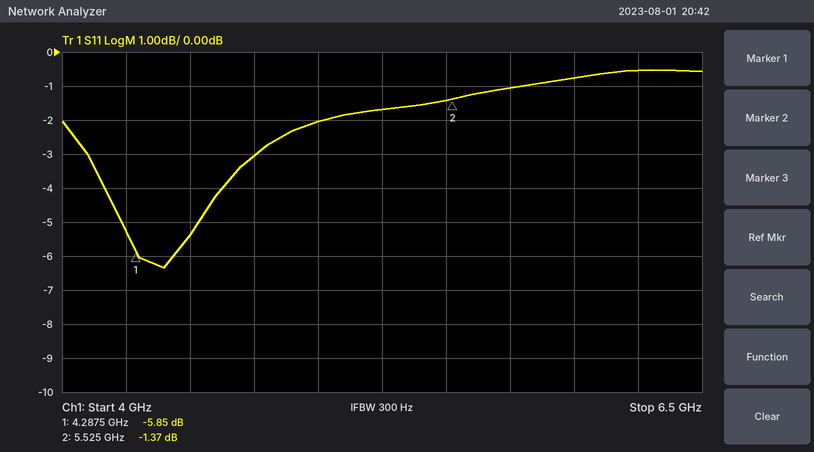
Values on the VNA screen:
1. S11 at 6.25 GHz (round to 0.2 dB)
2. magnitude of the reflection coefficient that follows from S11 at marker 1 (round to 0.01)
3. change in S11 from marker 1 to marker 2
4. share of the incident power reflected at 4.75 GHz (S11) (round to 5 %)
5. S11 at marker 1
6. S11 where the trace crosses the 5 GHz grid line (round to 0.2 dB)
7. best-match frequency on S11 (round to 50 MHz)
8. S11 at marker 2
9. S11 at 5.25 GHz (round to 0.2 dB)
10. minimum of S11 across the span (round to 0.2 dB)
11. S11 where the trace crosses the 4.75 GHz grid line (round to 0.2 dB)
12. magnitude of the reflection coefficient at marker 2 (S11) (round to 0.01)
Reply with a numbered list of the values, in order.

1. -0.6 dB
2. 0.51
3. 4.48 dB
4. 50 %
5. -5.85 dB
6. -2.0 dB
7. 4.40 GHz
8. -1.37 dB
9. -1.6 dB
10. -6.4 dB
11. -3.0 dB
12. 0.85
